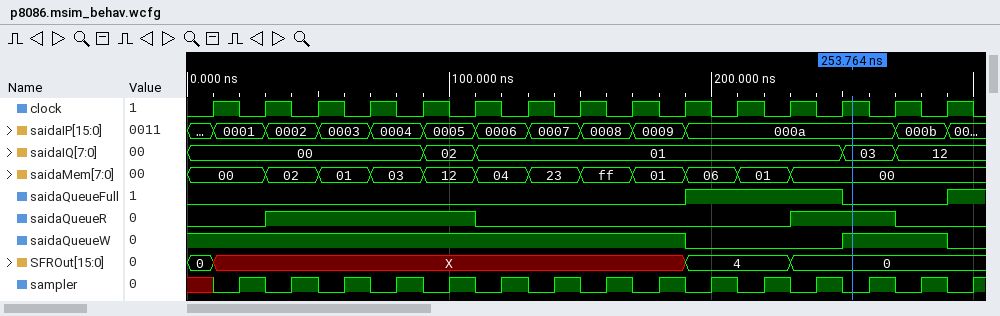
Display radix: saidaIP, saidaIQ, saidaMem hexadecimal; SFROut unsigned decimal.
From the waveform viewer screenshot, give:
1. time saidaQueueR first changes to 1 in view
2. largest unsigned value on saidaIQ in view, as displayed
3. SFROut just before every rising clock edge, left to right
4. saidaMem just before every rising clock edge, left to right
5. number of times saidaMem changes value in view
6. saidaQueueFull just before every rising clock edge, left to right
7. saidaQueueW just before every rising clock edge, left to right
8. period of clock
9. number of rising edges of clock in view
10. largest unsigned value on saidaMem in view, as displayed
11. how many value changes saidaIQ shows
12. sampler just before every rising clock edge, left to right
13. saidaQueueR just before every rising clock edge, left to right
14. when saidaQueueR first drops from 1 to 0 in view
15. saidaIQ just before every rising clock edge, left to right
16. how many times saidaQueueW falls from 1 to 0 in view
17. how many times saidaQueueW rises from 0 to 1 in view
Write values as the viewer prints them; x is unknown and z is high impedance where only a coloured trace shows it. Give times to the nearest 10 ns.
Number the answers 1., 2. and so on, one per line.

1. 30 ns
2. 12
3. 0, X, X, X, X, X, X, X, X, X, 4, 4, 0, 0, 0
4. 00, 00, 02, 01, 03, 12, 04, 23, ff, 01, 06, 01, 00, 00, 00
5. 11
6. 0 0 0 0 0 0 0 0 0 0 1 1 1 0 0
7. 1 1 1 1 1 1 1 1 1 1 0 0 0 1 1
8. 20 ns
9. 15
10. ff
11. 4
12. x 1 1 1 1 1 1 1 1 1 1 1 1 1 1
13. 0 0 1 1 1 1 0 0 0 0 0 0 1 1 0
14. 110 ns
15. 00, 00, 00, 00, 00, 02, 01, 01, 01, 01, 01, 01, 01, 03, 12
16. 2
17. 1
